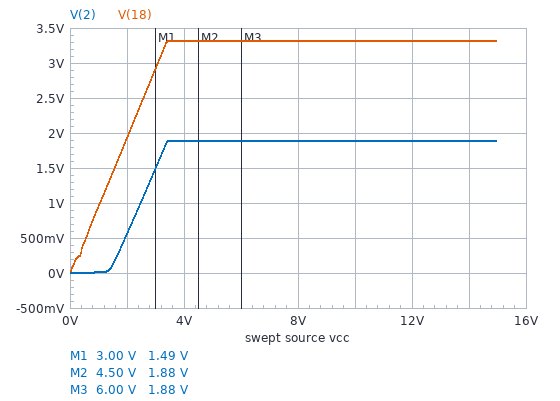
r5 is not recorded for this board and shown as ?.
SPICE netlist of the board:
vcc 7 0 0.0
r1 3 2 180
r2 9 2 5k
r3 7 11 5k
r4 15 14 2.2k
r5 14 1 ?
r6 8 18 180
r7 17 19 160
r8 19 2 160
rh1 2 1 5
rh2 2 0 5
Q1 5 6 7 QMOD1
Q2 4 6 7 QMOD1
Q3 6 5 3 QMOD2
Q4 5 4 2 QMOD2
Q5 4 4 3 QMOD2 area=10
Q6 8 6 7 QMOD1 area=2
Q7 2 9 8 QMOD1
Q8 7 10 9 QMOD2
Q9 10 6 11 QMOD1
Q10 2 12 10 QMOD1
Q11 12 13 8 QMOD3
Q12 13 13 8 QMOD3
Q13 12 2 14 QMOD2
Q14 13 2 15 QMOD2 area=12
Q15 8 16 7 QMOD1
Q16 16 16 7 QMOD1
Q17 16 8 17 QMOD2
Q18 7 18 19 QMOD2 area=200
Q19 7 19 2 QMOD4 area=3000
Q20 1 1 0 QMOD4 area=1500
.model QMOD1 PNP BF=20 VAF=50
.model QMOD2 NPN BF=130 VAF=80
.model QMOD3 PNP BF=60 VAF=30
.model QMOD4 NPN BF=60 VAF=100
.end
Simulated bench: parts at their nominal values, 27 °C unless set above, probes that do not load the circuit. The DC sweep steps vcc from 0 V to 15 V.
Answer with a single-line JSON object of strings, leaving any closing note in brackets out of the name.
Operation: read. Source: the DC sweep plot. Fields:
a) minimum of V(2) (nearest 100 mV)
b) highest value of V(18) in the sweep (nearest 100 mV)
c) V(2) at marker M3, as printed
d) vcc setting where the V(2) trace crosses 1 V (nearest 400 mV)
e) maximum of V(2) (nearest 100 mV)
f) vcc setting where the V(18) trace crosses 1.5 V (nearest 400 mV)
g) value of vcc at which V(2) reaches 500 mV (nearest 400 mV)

{"minimum of V(2)": "0 V", "highest value of V(18) in the sweep": "3.3 V", "V(2) at marker M3, as printed": "1.88 V", "vcc setting where the V(2) trace crosses 1 V": "2.4 V", "maximum of V(2)": "1.9 V", "vcc setting where the V(18) trace crosses 1.5 V": "1.6 V", "value of vcc at which V(2) reaches 500 mV": "2.0 V"}
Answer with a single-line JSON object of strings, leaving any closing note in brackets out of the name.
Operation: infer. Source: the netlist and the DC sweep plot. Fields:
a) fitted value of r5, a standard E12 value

{"fitted value of r5, a standard E12 value": "8.2 kΩ"}
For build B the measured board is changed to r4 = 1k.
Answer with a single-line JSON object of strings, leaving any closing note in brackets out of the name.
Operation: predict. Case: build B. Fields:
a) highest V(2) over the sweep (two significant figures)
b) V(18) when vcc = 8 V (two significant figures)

{"highest V(2) over the sweep": "2.5 V", "V(18) when vcc = 8 V": "3.9 V"}
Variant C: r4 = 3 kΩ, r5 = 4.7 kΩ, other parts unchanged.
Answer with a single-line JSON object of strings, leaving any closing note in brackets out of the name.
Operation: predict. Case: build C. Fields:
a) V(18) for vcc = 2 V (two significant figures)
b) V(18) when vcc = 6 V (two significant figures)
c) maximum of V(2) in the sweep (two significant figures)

{"V(18) for vcc = 2 V": "1.9 V", "V(18) when vcc = 6 V": "3.0 V", "maximum of V(2) in the sweep": "1.6 V"}
